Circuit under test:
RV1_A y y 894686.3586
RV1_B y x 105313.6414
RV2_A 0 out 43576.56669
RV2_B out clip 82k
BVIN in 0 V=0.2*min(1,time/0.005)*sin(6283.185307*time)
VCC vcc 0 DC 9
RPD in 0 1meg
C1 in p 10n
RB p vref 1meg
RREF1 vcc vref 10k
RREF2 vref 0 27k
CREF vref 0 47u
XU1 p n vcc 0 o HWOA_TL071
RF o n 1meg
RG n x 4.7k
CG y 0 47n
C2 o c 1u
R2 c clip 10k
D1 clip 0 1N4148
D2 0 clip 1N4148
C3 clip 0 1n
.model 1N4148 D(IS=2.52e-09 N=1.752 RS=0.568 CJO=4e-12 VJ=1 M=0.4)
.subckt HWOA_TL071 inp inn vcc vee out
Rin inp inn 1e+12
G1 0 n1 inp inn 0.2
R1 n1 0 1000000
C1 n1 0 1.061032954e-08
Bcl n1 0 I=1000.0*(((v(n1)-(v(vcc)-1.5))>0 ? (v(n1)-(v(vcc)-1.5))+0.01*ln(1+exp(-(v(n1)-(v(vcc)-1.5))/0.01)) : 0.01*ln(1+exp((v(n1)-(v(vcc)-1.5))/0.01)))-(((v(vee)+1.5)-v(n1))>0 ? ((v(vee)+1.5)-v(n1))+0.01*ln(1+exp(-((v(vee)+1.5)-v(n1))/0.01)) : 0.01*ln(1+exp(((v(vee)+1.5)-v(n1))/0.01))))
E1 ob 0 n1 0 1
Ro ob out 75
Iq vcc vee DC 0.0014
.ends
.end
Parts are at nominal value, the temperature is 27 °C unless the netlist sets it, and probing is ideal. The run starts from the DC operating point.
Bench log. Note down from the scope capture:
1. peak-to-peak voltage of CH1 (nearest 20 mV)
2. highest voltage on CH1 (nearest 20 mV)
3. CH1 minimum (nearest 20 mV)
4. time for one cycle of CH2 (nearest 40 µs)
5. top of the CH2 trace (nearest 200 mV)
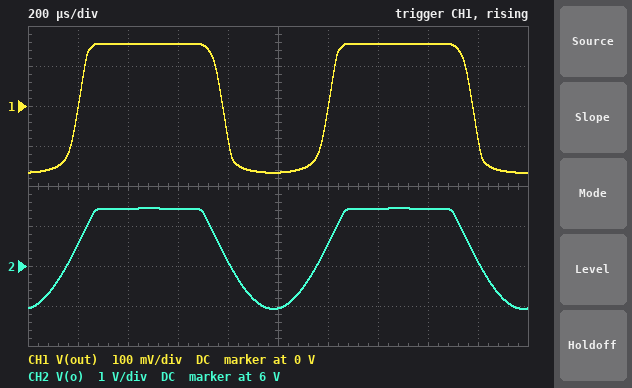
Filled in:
320 mV
160 mV
-160 mV
1.00 ms
7.4 V
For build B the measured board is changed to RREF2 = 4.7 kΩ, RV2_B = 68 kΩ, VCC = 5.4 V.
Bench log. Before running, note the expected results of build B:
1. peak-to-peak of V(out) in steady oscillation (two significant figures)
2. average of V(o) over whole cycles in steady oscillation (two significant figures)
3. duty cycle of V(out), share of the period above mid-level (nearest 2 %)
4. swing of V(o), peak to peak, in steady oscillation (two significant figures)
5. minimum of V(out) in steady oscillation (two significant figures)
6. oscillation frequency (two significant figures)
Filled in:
300 mV
1.8 V
28 %
1.2 V
-140 mV
1.0 kHz
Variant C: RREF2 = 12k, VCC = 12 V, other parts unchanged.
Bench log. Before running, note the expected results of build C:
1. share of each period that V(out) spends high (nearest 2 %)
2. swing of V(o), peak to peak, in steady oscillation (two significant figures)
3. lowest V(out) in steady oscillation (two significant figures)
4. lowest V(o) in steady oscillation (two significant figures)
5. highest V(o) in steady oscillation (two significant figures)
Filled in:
50 %
4.0 V
-170 mV
4.5 V
8.6 V
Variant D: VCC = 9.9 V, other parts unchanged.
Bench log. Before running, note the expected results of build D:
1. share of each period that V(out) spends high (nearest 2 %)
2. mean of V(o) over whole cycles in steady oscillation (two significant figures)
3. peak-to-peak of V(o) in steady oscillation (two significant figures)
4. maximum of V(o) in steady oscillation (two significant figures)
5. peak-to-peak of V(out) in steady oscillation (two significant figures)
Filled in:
56 %
7.2 V
2.9 V
8.3 V
330 mV
